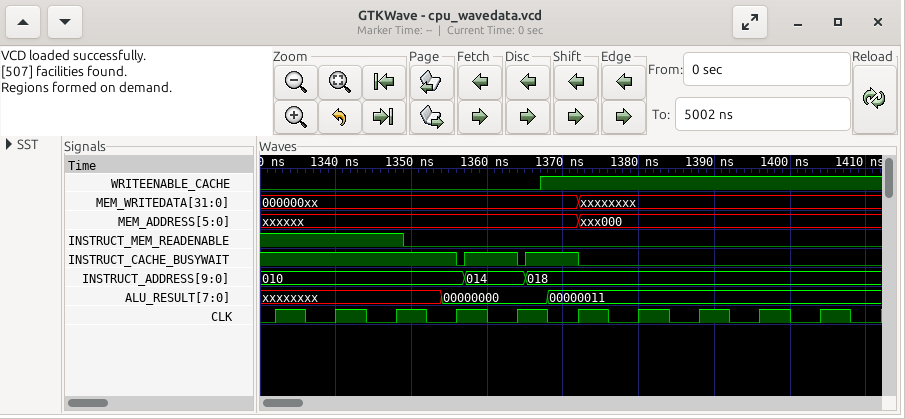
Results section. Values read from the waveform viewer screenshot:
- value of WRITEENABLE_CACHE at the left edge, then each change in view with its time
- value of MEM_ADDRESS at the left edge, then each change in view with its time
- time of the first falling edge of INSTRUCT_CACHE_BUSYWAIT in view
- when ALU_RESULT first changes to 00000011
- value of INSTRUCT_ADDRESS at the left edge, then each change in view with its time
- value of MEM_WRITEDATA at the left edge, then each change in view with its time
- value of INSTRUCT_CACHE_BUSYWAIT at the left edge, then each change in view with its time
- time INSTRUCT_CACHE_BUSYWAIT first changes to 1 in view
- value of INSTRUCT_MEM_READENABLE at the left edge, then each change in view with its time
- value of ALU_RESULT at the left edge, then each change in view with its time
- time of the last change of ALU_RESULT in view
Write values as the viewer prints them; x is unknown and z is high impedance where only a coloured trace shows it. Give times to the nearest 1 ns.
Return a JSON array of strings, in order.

["0, 1 at 1367 ns", "xxxxxx, xxx000 at 1372 ns", "1356 ns", "1368 ns", "010, 014 at 1357 ns, 018 at 1365 ns", "000000xx, xxxxxxxx at 1372 ns", "1, 0 at 1356 ns, 1 at 1357 ns, 0 at 1364 ns, 1 at 1365 ns, 0 at 1372 ns", "1357 ns", "1, 0 at 1349 ns", "xxxxxxxx, 00000000 at 1354 ns, 00000011 at 1368 ns", "1368 ns"]
